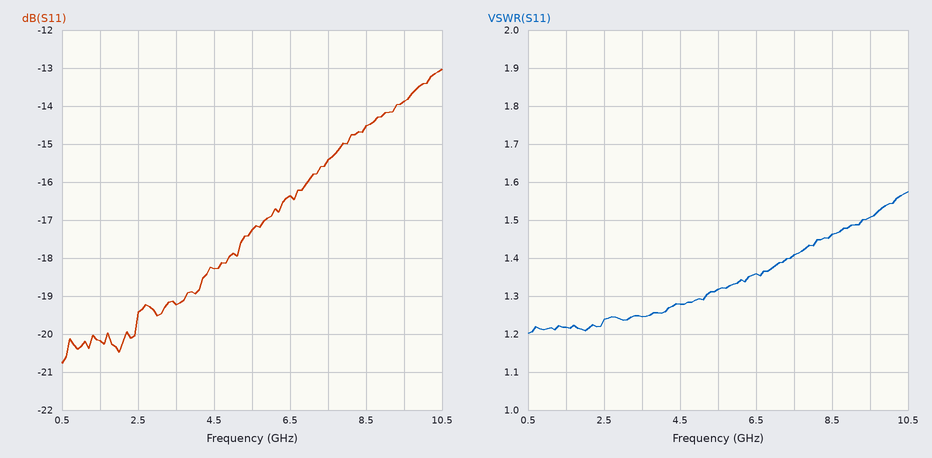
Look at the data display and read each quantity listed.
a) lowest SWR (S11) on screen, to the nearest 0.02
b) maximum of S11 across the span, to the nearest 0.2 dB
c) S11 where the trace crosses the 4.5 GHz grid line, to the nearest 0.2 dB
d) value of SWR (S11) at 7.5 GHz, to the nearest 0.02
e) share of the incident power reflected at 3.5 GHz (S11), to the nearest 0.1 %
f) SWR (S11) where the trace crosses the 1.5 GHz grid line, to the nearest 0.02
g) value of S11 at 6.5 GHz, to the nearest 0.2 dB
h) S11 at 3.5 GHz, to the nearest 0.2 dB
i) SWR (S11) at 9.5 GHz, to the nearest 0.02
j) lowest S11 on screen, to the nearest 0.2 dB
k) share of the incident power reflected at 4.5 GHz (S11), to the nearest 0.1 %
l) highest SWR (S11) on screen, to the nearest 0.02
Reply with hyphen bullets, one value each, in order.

- 1.20
- -13.0 dB
- -18.2 dB
- 1.40
- 1.2 %
- 1.22
- -16.4 dB
- -19.2 dB
- 1.50
- -20.8 dB
- 1.5 %
- 1.58
